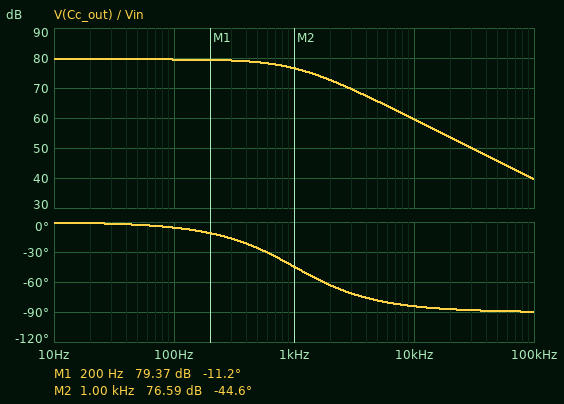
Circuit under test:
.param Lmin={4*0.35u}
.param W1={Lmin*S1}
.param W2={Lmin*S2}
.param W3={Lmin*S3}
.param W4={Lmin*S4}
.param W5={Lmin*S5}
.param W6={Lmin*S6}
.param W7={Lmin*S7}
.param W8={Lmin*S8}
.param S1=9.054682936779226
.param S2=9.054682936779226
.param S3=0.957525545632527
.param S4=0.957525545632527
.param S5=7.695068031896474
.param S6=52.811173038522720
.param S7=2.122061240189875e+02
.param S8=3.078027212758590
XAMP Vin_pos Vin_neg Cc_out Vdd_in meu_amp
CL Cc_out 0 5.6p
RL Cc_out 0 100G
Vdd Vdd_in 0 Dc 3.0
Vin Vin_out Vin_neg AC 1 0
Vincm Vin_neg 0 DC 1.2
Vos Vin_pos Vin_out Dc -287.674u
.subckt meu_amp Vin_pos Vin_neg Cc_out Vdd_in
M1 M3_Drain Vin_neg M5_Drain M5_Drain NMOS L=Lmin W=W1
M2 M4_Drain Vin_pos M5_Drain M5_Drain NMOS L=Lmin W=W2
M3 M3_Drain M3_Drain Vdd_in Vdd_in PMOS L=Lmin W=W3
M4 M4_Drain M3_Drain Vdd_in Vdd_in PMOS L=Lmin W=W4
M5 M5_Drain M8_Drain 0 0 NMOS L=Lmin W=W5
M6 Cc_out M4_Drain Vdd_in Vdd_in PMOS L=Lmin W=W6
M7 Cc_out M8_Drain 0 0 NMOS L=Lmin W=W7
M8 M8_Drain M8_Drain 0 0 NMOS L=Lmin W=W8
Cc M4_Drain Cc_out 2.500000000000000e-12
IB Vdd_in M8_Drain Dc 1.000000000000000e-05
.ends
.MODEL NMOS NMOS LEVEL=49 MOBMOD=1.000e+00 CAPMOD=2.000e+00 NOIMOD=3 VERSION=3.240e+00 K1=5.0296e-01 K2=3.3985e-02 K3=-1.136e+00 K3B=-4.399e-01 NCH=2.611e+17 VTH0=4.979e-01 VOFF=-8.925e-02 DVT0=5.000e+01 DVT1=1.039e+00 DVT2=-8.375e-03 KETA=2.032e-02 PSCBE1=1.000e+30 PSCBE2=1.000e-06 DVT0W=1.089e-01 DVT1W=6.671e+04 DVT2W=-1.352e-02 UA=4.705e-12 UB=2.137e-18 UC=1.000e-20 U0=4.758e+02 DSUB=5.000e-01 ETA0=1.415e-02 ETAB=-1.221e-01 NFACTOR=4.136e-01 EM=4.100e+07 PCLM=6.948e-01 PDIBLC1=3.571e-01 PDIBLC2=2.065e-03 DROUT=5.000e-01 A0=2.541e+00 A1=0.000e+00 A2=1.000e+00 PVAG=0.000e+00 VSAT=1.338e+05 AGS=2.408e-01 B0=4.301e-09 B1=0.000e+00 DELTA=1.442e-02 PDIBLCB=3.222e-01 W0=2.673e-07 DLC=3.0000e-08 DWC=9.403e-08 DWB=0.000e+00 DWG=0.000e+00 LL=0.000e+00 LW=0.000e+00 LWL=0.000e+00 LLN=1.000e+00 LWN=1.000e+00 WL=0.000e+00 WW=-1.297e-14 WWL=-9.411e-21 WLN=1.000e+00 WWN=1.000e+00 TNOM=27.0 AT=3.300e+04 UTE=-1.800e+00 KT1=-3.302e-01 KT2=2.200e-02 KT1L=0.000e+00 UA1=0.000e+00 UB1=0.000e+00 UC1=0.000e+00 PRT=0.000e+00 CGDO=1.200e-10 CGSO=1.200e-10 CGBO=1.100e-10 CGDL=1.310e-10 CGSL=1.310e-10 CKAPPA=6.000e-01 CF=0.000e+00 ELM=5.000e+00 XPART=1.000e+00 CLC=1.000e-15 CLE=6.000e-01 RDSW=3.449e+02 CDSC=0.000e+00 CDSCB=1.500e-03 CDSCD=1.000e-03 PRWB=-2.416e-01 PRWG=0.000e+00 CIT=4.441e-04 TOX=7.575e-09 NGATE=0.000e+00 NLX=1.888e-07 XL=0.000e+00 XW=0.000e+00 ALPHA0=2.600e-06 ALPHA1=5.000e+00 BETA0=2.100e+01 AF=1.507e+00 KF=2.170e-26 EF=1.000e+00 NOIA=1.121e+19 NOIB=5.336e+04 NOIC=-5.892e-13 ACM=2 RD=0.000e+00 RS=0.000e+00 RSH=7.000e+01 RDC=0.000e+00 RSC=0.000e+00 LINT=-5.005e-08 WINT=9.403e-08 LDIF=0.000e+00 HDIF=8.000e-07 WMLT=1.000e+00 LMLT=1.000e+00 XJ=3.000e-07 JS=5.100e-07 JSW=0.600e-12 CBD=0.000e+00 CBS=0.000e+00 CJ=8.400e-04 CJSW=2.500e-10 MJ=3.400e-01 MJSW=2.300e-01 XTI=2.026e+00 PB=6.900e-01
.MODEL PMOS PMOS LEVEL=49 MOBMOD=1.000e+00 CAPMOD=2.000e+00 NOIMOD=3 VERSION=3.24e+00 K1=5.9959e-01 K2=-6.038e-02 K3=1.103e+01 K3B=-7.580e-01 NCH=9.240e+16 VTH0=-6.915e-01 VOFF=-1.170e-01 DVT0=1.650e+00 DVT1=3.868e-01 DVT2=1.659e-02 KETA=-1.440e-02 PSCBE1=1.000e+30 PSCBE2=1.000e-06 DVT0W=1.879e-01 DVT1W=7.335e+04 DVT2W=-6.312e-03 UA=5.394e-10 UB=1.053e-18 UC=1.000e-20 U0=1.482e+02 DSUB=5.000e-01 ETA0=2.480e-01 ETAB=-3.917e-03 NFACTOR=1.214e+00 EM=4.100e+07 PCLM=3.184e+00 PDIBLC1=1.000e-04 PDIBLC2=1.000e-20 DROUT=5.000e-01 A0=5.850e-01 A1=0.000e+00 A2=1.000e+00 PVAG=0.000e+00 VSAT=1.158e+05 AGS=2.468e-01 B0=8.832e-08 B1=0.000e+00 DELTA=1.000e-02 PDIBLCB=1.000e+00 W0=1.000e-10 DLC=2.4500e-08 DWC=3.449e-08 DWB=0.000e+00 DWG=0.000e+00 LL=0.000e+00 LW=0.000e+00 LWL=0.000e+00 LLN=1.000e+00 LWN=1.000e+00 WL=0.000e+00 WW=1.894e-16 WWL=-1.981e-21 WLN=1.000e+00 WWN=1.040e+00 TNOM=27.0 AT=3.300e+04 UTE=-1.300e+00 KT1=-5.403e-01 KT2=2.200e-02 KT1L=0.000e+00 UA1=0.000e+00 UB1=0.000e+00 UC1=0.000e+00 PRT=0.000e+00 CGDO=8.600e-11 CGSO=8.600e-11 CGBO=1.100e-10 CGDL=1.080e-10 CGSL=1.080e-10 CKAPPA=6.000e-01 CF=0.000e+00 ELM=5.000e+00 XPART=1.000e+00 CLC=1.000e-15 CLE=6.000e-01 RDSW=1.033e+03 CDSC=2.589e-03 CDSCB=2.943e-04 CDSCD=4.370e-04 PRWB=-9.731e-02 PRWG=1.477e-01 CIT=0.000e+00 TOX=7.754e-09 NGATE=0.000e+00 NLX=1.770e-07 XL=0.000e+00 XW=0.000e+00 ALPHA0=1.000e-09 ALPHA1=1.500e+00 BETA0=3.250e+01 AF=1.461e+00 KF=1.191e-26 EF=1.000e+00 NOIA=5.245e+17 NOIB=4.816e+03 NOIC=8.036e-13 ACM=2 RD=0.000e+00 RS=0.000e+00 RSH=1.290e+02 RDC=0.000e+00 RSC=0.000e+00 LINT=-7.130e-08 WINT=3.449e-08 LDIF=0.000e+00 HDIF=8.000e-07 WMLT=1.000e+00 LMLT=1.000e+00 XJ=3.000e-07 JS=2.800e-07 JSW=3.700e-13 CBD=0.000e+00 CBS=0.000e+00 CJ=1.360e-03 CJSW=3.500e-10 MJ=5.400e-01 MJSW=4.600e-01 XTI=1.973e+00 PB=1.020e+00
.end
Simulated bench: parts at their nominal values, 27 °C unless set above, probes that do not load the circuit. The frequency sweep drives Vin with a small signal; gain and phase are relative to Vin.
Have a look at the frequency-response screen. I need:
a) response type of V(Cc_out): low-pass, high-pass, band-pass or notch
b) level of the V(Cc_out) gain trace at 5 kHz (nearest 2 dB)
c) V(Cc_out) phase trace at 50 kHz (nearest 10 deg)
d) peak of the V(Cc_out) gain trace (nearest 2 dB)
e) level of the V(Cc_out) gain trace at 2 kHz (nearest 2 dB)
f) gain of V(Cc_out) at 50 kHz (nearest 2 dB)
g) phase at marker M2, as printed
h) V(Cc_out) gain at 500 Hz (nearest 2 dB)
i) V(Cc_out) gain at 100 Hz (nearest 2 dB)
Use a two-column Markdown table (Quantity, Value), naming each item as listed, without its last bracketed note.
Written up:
| Quantity | Value |
|---|---|
| response type of V(Cc_out): low-pass, high-pass, band-pass or notch | low-pass |
| level of the V(Cc_out) gain trace at 5 kHz | 66 dB |
| V(Cc_out) phase trace at 50 kHz | -90 deg |
| peak of the V(Cc_out) gain trace | 80 dB |
| level of the V(Cc_out) gain trace at 2 kHz | 72 dB |
| gain of V(Cc_out) at 50 kHz | 46 dB |
| phase at marker M2, as printed | -44.6 deg |
| V(Cc_out) gain at 500 Hz | 78 dB |
| V(Cc_out) gain at 100 Hz | 80 dB |
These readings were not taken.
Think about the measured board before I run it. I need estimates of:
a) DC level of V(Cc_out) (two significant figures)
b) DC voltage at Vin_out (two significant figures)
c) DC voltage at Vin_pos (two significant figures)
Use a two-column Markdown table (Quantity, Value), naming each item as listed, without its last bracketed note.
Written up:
| Quantity | Value |
|---|---|
| DC level of V(Cc_out) | 1.5 V |
| DC voltage at Vin_out | 1.2 V |
| DC voltage at Vin_pos | 1.2 V |
